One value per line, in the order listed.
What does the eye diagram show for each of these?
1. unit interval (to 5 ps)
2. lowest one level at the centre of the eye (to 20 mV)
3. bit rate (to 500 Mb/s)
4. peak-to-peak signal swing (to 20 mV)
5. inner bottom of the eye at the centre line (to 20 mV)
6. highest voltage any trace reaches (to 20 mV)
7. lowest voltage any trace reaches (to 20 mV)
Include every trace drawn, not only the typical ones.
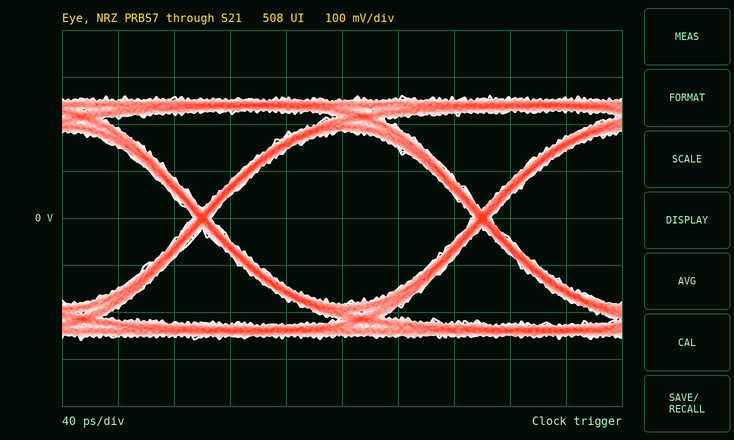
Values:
200 ps
180 mV
5.0 Gb/s
520 mV
-180 mV
260 mV
-260 mV
